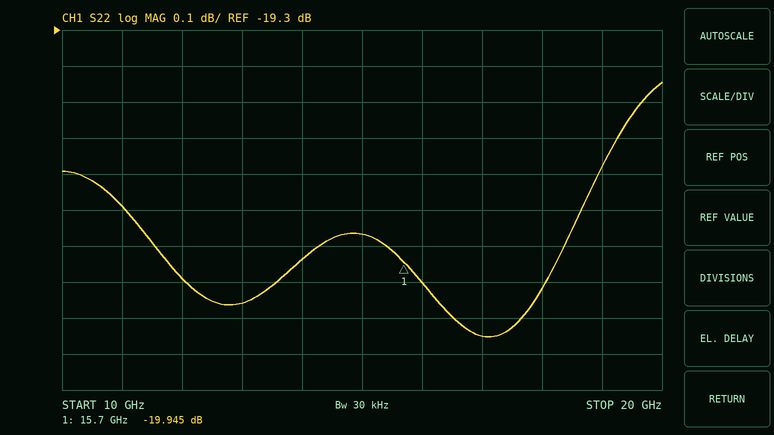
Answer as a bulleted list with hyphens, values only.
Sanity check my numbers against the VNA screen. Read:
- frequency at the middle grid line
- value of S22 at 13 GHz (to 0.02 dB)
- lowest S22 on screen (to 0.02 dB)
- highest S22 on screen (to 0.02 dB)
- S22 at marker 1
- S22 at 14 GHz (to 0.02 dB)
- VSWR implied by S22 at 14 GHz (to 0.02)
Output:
- 15 GHz
- -20.06 dB
- -20.16 dB
- -19.44 dB
- -19.945 dB
- -19.94 dB
- 1.22
